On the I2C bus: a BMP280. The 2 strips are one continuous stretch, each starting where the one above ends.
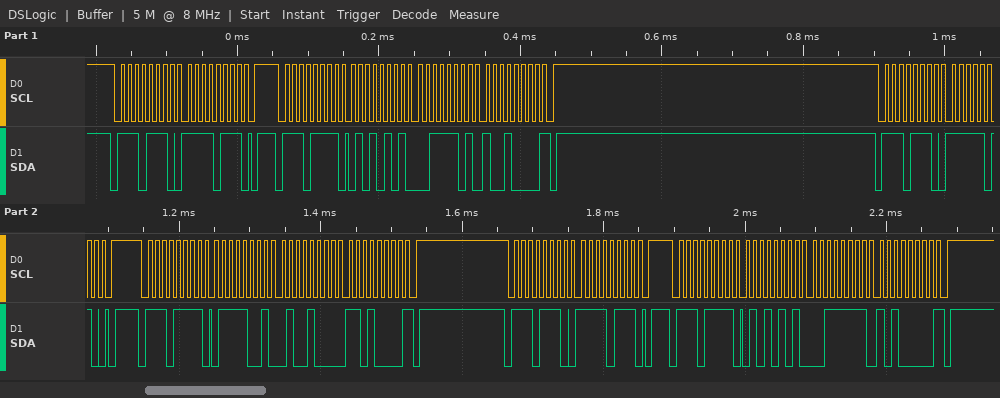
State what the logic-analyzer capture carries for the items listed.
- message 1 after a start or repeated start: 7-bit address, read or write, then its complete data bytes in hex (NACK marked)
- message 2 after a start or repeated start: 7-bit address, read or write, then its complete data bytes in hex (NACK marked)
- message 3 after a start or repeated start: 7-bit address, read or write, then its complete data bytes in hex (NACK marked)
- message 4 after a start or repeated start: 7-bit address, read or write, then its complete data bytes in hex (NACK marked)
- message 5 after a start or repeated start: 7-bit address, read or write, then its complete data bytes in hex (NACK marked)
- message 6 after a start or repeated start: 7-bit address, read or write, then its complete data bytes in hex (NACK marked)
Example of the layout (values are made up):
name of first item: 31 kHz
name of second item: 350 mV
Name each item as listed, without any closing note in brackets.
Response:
message 1 after a start or repeated start: 7-bit address, read or write, then its complete data bytes in hex: 0x77 write: F7
message 2 after a start or repeated start: 7-bit address, read or write, then its complete data bytes in hex: 0x77 read: 55 3D 90 NACK
message 3 after a start or repeated start: 7-bit address, read or write, then its complete data bytes in hex: 0x77 write: FA
message 4 after a start or repeated start: 7-bit address, read or write, then its complete data bytes in hex: 0x77 read: 79 48 D0 NACK
message 5 after a start or repeated start: 7-bit address, read or write, then its complete data bytes in hex: 0x77 write: F7
message 6 after a start or repeated start: 7-bit address, read or write, then its complete data bytes in hex: 0x77 read: 55 3F A0 NACK
